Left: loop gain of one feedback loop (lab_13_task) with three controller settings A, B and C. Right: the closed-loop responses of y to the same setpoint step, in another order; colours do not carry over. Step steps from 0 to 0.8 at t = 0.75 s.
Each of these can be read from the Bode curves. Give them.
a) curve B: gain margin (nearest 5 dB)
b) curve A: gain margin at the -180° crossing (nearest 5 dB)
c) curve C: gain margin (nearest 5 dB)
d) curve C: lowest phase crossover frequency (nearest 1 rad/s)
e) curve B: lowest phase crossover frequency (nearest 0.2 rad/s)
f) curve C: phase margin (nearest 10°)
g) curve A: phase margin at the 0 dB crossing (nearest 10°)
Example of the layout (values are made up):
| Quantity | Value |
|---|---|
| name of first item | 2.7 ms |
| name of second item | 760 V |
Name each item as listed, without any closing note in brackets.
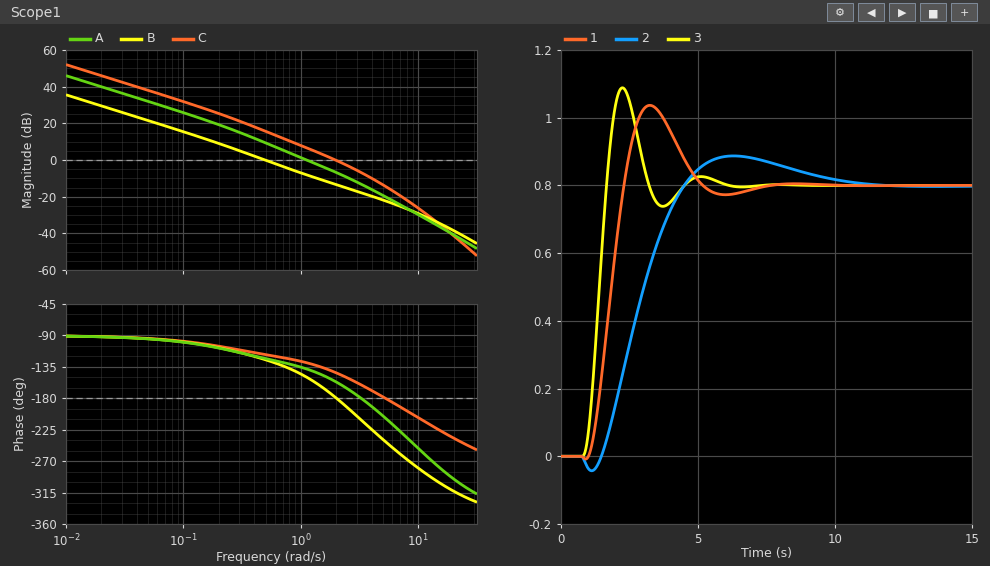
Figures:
| Quantity | Value |
|---|---|
| curve B: gain margin | 15 dB |
| curve A: gain margin at the -180° crossing | 15 dB |
| curve C: gain margin | 15 dB |
| curve C: lowest phase crossover frequency | 5 rad/s |
| curve B: lowest phase crossover frequency | 2.0 rad/s |
| curve C: phase margin | 40° |
| curve A: phase margin at the 0 dB crossing | 40° |
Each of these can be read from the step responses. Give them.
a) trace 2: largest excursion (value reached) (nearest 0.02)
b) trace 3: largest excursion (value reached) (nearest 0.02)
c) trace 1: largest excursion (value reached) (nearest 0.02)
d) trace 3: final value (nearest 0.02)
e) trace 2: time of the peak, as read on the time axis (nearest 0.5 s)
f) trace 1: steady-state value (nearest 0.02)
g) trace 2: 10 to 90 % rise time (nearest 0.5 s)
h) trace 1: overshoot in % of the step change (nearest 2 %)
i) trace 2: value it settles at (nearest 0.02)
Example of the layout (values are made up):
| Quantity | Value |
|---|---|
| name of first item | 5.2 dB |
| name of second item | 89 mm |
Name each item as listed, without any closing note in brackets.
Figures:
| Quantity | Value |
|---|---|
| trace 2: largest excursion (value reached) | 0.88 |
| trace 3: largest excursion (value reached) | 1.08 |
| trace 1: largest excursion (value reached) | 1.04 |
| trace 3: final value | 0.80 |
| trace 2: time of the peak, as read on the time axis | 6.5 s |
| trace 1: steady-state value | 0.80 |
| trace 2: 10 to 90 % rise time | 2.0 s |
| trace 1: overshoot in % of the step change | 30 % |
| trace 2: value it settles at | 0.80 |
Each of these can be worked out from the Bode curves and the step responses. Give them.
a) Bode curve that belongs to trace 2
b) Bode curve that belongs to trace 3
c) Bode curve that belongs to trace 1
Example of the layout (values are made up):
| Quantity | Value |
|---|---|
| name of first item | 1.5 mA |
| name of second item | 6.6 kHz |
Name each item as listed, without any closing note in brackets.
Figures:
| Quantity | Value |
|---|---|
| Bode curve that belongs to trace 2 | B |
| Bode curve that belongs to trace 3 | C |
| Bode curve that belongs to trace 1 | A |
